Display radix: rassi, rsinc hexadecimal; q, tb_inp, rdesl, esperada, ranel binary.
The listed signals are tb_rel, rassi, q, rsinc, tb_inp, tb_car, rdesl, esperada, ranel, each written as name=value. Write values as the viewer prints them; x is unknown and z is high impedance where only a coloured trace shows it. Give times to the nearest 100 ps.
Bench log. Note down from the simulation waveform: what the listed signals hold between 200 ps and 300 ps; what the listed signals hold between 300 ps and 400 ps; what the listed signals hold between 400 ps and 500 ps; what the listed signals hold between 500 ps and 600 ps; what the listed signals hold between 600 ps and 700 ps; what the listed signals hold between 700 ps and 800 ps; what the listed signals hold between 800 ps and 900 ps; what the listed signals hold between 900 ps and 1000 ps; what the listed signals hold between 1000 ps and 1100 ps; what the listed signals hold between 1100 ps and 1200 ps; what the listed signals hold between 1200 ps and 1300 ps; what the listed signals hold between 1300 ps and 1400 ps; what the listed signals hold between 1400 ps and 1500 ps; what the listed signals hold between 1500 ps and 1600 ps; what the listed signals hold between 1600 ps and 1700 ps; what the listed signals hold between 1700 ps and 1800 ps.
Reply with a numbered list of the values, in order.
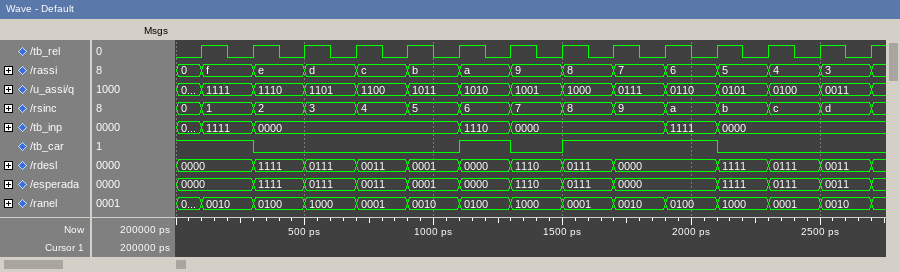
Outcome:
1. tb_rel=0, rassi=f, q=1111, rsinc=1, tb_inp=1111, tb_car=1, rdesl=0000, esperada=0000, ranel=0010
2. tb_rel=1, rassi=e, q=1110, rsinc=2, tb_inp=0000, tb_car=0, rdesl=1111, esperada=1111, ranel=0100
3. tb_rel=0, rassi=e, q=1110, rsinc=2, tb_inp=0000, tb_car=0, rdesl=1111, esperada=1111, ranel=0100
4. tb_rel=1, rassi=d, q=1101, rsinc=3, tb_inp=0000, tb_car=0, rdesl=0111, esperada=0111, ranel=1000
5. tb_rel=0, rassi=d, q=1101, rsinc=3, tb_inp=0000, tb_car=0, rdesl=0111, esperada=0111, ranel=1000
6. tb_rel=1, rassi=c, q=1100, rsinc=4, tb_inp=0000, tb_car=0, rdesl=0011, esperada=0011, ranel=0001
7. tb_rel=0, rassi=c, q=1100, rsinc=4, tb_inp=0000, tb_car=0, rdesl=0011, esperada=0011, ranel=0001
8. tb_rel=1, rassi=b, q=1011, rsinc=5, tb_inp=0000, tb_car=0, rdesl=0001, esperada=0001, ranel=0010
9. tb_rel=0, rassi=b, q=1011, rsinc=5, tb_inp=0000, tb_car=0, rdesl=0001, esperada=0001, ranel=0010
10. tb_rel=1, rassi=a, q=1010, rsinc=6, tb_inp=1110, tb_car=1, rdesl=0000, esperada=0000, ranel=0100
11. tb_rel=0, rassi=a, q=1010, rsinc=6, tb_inp=1110, tb_car=1, rdesl=0000, esperada=0000, ranel=0100
12. tb_rel=1, rassi=9, q=1001, rsinc=7, tb_inp=0000, tb_car=0, rdesl=1110, esperada=1110, ranel=1000
13. tb_rel=0, rassi=9, q=1001, rsinc=7, tb_inp=0000, tb_car=0, rdesl=1110, esperada=1110, ranel=1000
14. tb_rel=1, rassi=8, q=1000, rsinc=8, tb_inp=0000, tb_car=1, rdesl=0111, esperada=0111, ranel=0001
15. tb_rel=0, rassi=8, q=1000, rsinc=8, tb_inp=0000, tb_car=1, rdesl=0111, esperada=0111, ranel=0001
16. tb_rel=1, rassi=7, q=0111, rsinc=9, tb_inp=0000, tb_car=1, rdesl=0000, esperada=0000, ranel=0010
